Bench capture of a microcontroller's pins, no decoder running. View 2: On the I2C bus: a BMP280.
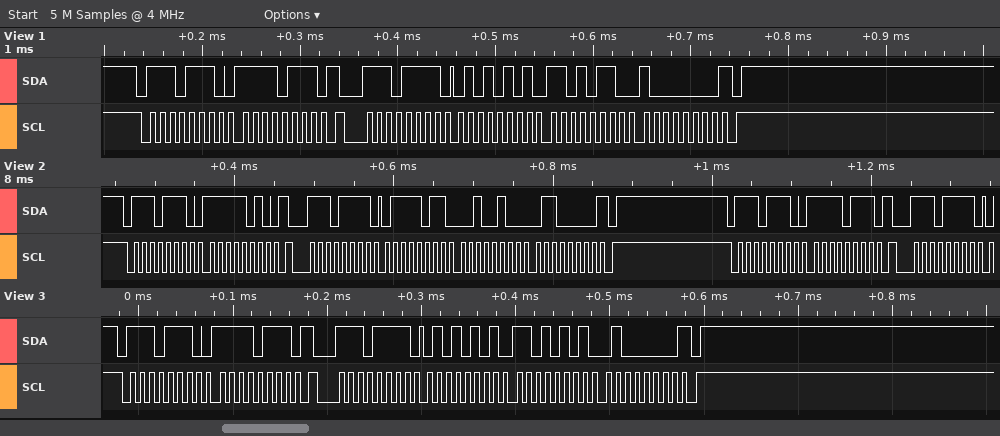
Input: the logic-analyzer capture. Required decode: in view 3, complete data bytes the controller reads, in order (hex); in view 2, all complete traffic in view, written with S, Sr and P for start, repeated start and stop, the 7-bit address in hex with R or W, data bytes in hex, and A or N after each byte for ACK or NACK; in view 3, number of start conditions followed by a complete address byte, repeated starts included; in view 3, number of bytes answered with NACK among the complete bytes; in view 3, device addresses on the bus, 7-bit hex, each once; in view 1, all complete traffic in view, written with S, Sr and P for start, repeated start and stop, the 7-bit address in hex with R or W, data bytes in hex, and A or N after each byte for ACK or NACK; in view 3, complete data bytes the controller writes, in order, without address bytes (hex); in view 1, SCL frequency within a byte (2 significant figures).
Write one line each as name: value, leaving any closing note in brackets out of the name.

in view 3, complete data bytes the controller reads, in order: 55 D5 40
in view 2, all complete traffic in view, written with S, Sr and P for start, repeated start and stop, the 7-bit address in hex with R or W, data bytes in hex, and A or N after each byte for ACK or NACK: S 77W A FA A Sr 77R A 7B A 24 A 60 N P S 77W A F7 A Sr 77R A
in view 3, number of start conditions followed by a complete address byte, repeated starts included: 2
in view 3, number of bytes answered with NACK among the complete bytes: 1
in view 3, device addresses on the bus, 7-bit hex, each once: 0x77
in view 1, all complete traffic in view, written with S, Sr and P for start, repeated start and stop, the 7-bit address in hex with R or W, data bytes in hex, and A or N after each byte for ACK or NACK: S 77W A F7 A Sr 77R A 55 A D6 A 80 N P
in view 3, complete data bytes the controller writes, in order, without address bytes: F7
in view 1, SCL frequency within a byte: 100 kHz
